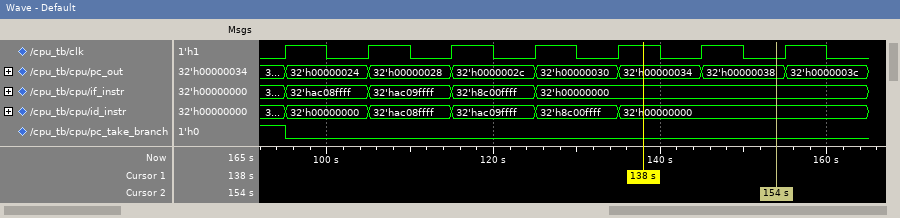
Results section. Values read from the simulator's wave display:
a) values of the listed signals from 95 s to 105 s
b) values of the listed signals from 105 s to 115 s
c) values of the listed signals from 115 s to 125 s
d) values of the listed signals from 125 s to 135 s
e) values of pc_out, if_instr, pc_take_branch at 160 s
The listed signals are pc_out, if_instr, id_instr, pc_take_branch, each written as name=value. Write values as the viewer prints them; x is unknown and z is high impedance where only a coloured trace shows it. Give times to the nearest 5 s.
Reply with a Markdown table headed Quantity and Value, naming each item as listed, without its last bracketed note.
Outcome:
| Quantity | Value |
|---|---|
| values of the listed signals from 95 s to 105 s | pc_out=32'h00000024, if_instr=32'hac08ffff, id_instr=32'h00000000, pc_take_branch=0 |
| values of the listed signals from 105 s to 115 s | pc_out=32'h00000028, if_instr=32'hac09ffff, id_instr=32'hac08ffff, pc_take_branch=0 |
| values of the listed signals from 115 s to 125 s | pc_out=32'h0000002c, if_instr=32'h8c00ffff, id_instr=32'hac09ffff, pc_take_branch=0 |
| values of the listed signals from 125 s to 135 s | pc_out=32'h00000030, if_instr=32'h00000000, id_instr=32'h8c00ffff, pc_take_branch=0 |
| values of pc_out, if_instr, pc_take_branch at 160 s | pc_out=32'h0000003c, if_instr=32'h00000000, pc_take_branch=0 |
